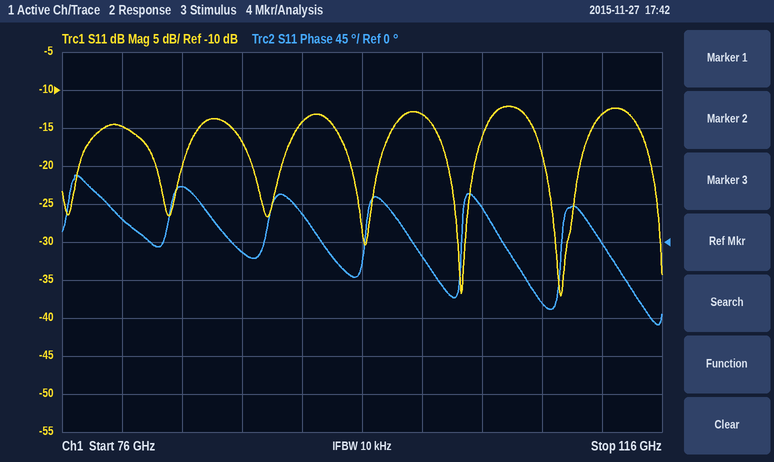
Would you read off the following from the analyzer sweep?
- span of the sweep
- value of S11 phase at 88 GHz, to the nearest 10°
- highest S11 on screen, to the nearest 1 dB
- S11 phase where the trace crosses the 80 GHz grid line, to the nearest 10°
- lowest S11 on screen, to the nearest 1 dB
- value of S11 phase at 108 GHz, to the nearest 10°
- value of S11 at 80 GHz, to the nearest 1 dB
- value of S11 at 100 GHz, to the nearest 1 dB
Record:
40 GHz
-10°
-12 dB
30°
-37 dB
-70°
-15 dB
-13 dB
